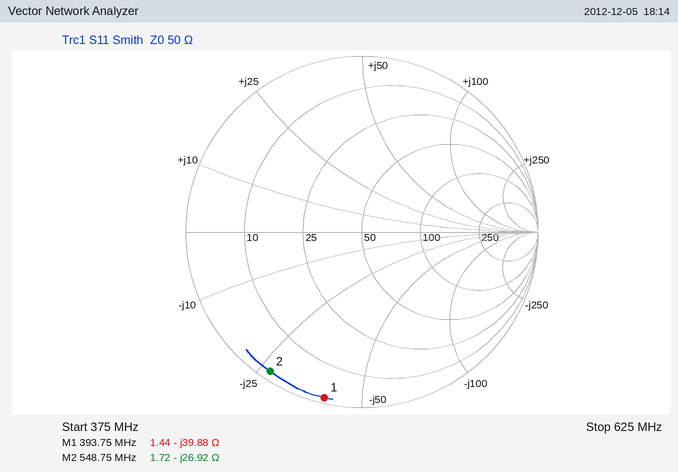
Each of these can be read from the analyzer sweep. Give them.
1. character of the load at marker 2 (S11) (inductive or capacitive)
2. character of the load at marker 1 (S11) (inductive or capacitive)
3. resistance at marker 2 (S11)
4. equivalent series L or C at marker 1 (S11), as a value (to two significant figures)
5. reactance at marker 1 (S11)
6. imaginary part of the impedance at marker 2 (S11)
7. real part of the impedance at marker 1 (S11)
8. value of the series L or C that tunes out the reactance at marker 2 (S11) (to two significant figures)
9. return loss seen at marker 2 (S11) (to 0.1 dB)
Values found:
capacitive
capacitive
1.72 Ω
10 pF
-39.88 Ω
-26.92 Ω
1.44 Ω
7.8 nH
0.5 dB
